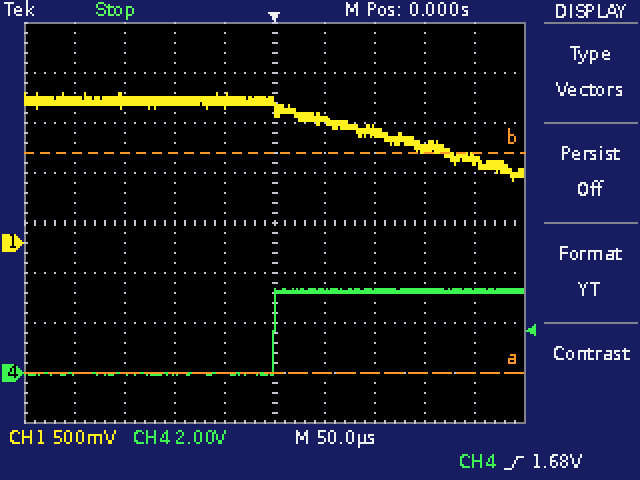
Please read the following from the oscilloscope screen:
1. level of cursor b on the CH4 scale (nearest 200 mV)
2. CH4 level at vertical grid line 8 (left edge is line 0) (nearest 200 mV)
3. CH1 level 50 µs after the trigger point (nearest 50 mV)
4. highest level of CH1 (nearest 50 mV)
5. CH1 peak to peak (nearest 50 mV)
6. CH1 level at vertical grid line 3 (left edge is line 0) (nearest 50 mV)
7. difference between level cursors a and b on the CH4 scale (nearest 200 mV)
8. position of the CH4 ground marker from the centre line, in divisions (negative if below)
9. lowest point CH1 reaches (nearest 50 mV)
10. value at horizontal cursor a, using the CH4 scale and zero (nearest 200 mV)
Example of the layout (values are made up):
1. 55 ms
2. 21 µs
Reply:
1. 8.8 V
2. 3.2 V
3. 1.20 V
4. 1.50 V
5. 900 mV
6. 1.40 V
7. 8.8 V
8. -3.0 div
9. 600 mV
10. 0.0 V
